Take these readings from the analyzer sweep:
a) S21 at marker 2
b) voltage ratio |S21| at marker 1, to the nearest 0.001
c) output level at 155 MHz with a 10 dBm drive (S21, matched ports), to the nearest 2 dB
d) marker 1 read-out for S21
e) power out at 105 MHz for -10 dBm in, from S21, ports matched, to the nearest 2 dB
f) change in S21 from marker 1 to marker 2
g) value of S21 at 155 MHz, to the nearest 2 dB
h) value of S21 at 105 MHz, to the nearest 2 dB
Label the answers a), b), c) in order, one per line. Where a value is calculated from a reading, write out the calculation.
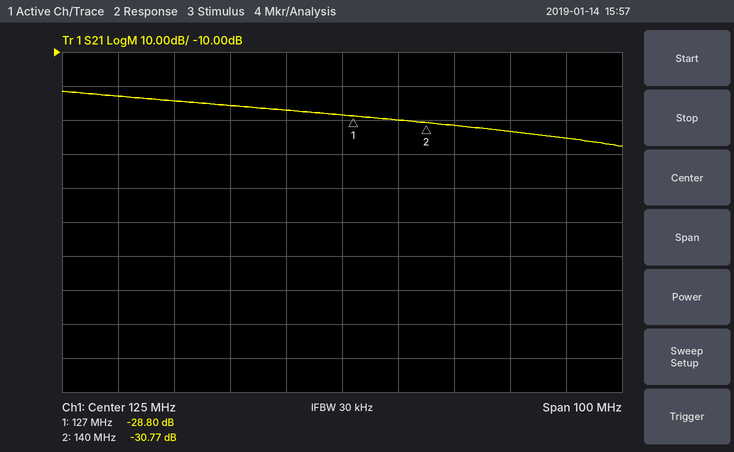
a) -30.77 dB
b) 10^(-28.8/20) ≈ 0.036
c) 10 dBm + (-34 dB) = -24 dBm
d) -28.80 dB
e) -10 dBm + (-26 dB) = -36 dBm
f) -30.77 − (-28.8) = -1.97 dB
g) -34 dB
h) -26 dB
